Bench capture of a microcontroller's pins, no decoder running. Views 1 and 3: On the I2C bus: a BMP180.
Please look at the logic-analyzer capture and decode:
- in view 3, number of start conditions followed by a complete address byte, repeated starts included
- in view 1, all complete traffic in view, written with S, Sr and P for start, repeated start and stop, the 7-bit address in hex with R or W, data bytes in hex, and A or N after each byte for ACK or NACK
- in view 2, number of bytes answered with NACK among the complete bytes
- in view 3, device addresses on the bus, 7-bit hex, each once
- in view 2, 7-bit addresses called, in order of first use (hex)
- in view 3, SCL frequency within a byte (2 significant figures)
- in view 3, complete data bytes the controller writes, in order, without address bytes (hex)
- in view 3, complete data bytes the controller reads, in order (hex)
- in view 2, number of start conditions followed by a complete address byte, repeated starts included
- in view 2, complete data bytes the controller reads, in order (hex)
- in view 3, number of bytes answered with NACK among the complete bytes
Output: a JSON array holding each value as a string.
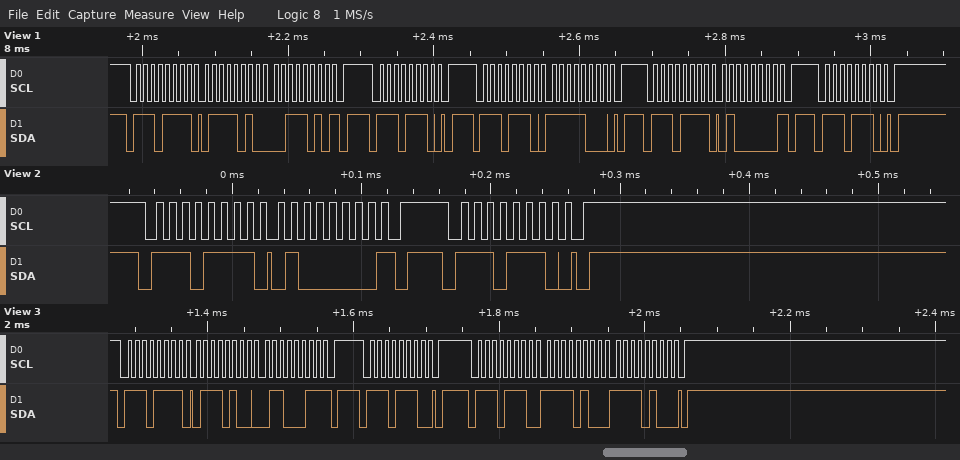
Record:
["3", "S 77R A 7A A 3A N P S 77W A P S 77W A F8 A P S 77R A 40 N P S 77W A P", "1", "0x77", "0x77", "100 kHz", "F4 F4", "74 63", "2", "40", "1"]
